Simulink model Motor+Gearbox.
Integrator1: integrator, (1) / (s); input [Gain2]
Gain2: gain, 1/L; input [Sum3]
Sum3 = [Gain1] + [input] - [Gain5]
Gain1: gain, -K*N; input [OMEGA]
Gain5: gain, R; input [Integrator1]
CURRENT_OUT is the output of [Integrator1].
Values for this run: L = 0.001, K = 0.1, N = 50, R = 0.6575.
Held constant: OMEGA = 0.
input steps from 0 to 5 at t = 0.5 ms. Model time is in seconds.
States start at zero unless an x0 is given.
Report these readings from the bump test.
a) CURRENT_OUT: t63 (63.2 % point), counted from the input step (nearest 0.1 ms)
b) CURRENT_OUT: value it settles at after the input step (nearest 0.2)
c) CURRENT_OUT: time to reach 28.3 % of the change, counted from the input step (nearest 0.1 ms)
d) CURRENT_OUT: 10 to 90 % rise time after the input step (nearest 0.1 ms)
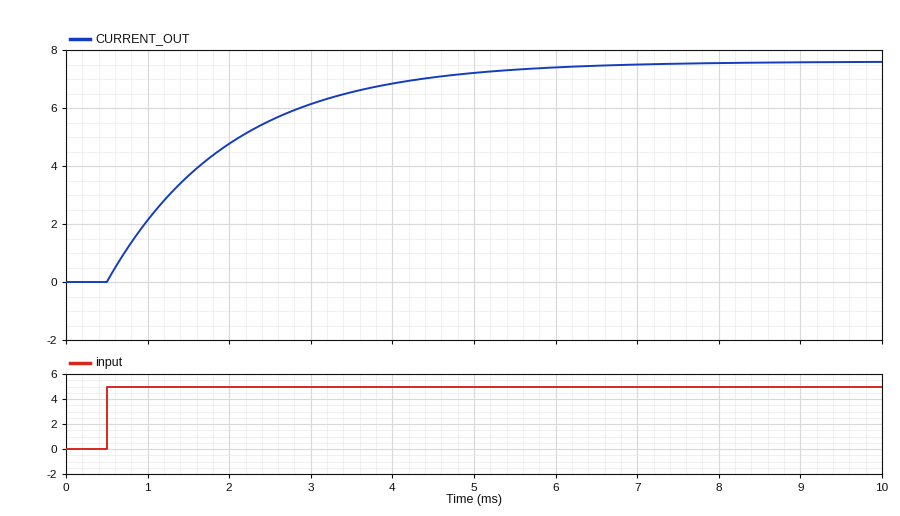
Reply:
1.5 ms
7.6
0.5 ms
3.3 ms
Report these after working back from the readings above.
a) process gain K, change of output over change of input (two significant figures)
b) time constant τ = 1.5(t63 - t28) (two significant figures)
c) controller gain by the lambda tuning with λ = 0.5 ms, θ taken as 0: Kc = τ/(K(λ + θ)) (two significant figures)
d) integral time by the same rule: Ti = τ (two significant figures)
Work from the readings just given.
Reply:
1.5
1.5 ms
2.0
1.5 ms
